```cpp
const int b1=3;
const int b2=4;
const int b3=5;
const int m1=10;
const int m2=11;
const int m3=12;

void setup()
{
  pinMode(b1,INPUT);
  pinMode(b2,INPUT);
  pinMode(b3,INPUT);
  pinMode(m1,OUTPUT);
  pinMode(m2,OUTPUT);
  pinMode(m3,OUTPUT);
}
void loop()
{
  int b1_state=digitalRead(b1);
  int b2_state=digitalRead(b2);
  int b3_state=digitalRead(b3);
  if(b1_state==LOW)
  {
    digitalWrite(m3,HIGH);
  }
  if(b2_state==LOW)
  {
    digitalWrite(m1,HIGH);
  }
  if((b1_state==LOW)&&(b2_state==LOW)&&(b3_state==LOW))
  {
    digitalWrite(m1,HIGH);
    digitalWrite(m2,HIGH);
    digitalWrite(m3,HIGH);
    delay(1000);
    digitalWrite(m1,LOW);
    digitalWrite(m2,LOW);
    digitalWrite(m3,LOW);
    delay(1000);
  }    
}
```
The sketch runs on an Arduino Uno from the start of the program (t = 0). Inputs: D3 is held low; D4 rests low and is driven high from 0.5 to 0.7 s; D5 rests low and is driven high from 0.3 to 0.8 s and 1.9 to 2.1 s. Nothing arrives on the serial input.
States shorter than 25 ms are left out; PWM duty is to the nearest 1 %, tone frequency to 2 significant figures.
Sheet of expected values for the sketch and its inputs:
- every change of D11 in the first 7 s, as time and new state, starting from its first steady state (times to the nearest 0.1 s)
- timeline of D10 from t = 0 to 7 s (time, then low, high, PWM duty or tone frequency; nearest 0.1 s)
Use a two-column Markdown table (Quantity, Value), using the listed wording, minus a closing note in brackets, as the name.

| Quantity | Value |
|---|---|
| every change of D11 in the first 7 s, as time and new state, starting from its first steady state | 0 s high; 1 s low; 2.1 s high; 3.1 s low; 4.1 s high; 5.1 s low; 6.1 s high |
| timeline of D10 from t = 0 to 7 s | 0 s high; 1 s low; 2 s high; 3.1 s low; 4.1 s high; 5.1 s low; 6.1 s high |
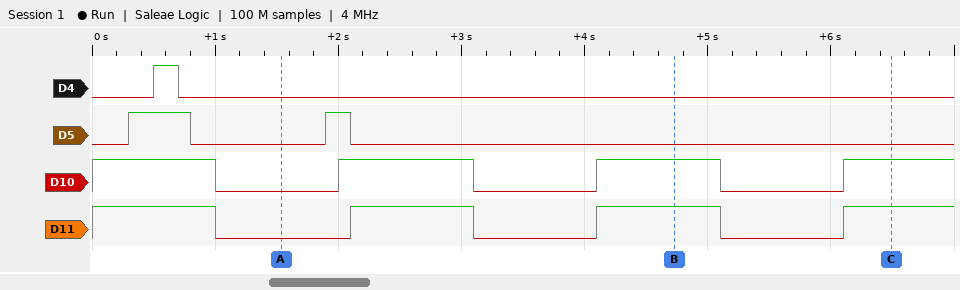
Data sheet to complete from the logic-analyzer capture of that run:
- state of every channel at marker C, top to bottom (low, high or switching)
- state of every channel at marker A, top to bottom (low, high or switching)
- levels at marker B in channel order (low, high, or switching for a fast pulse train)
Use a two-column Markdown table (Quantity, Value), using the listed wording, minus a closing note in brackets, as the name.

| Quantity | Value |
|---|---|
| state of every channel at marker C, top to bottom | D4 low, D5 low, D10 high, D11 high |
| state of every channel at marker A, top to bottom | D4 low, D5 low, D10 low, D11 low |
| levels at marker B in channel order | D4 low, D5 low, D10 high, D11 high |
